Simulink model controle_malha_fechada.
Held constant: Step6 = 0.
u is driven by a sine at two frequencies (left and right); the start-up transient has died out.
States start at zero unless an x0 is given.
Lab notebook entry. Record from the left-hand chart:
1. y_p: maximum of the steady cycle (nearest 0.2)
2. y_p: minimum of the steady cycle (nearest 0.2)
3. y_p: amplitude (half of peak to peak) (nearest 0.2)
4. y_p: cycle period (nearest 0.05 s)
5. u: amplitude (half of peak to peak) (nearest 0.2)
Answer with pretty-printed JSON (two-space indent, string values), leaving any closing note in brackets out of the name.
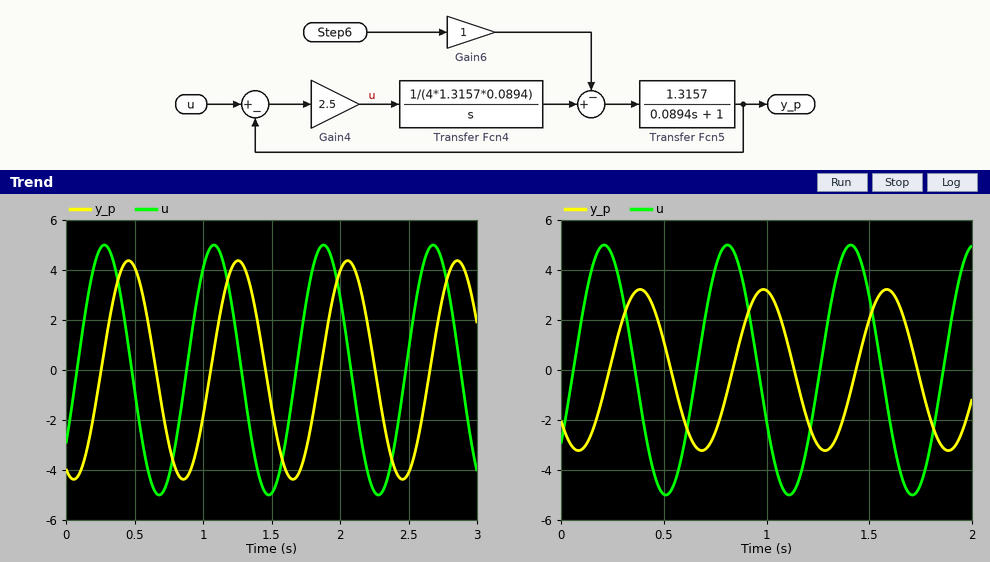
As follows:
{
  "y_p: maximum of the steady cycle": "4.4",
  "y_p: minimum of the steady cycle": "-4.4",
  "y_p: amplitude (half of peak to peak)": "4.4",
  "y_p: cycle period": "0.80 s",
  "u: amplitude (half of peak to peak)": "5.0"
}
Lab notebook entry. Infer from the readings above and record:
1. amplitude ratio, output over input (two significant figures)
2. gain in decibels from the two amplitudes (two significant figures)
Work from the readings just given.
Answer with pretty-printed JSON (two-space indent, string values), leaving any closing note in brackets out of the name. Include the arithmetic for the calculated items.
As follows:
{
  "amplitude ratio, output over input": "4.4 / 5 = 0.88",
  "gain in decibels from the two amplitudes": "20 log10(4.4 / 5) = -1.1 dB"
}
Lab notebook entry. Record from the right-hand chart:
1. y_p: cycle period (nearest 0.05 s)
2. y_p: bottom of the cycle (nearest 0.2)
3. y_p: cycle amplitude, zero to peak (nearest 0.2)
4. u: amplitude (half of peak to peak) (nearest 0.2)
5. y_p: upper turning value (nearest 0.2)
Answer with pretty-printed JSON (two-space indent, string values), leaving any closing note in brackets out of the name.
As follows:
{
  "y_p: cycle period": "0.60 s",
  "y_p: bottom of the cycle": "-3.2",
  "y_p: cycle amplitude, zero to peak": "3.2",
  "u: amplitude (half of peak to peak)": "5.0",
  "y_p: upper turning value": "3.2"
}
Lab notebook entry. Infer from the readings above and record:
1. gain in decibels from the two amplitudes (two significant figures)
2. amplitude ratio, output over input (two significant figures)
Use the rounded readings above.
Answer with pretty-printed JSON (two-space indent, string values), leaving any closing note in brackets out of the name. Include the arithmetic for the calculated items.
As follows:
{
  "gain in decibels from the two amplitudes": "20 log10(3.2 / 5) = -3.9 dB",
  "amplitude ratio, output over input": "3.2 / 5 = 0.64"
}
